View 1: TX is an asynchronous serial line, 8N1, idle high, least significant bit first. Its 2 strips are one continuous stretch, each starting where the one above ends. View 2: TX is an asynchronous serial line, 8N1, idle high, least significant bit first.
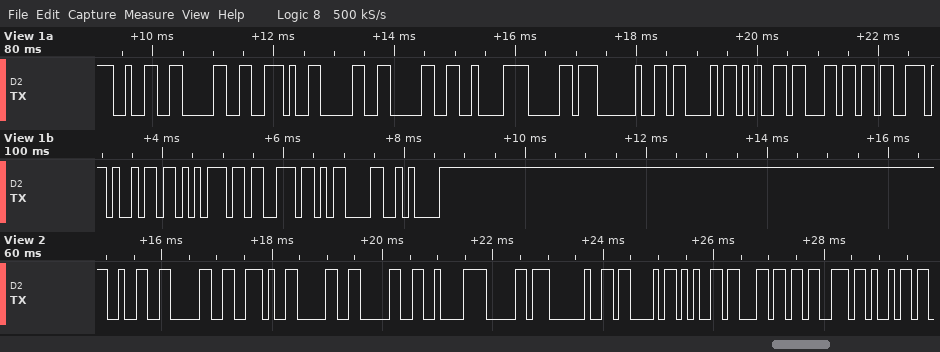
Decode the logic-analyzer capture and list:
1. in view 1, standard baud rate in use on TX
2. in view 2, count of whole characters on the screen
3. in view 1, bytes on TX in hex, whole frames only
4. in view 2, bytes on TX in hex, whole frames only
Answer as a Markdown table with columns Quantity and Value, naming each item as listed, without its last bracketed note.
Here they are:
| Quantity | Value |
|---|---|
| in view 1, standard baud rate in use on TX | 9600 baud |
| in view 2, count of whole characters on the screen | 13 |
| in view 1, bytes on TX in hex, whole frames only | 0x32 0x30 0x2E 0x30 0x30 0xC2 0xB0 0x20 0x43 0x65 0x6C 0x73 0x69 0x75 0x73 0x0D 0x0A |
| in view 2, bytes on TX in hex, whole frames only | 32 30 2E 30 30 C2 B0 20 43 65 6C 73 69 |
